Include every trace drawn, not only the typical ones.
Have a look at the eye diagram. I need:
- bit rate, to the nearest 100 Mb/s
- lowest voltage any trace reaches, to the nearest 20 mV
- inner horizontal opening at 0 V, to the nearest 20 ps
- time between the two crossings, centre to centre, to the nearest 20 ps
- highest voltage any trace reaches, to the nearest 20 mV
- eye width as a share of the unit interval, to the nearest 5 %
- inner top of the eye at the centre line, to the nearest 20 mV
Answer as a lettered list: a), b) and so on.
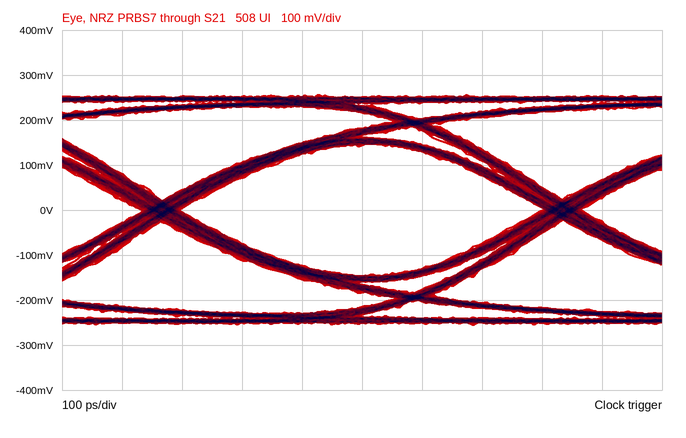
a) 1.5 Gb/s
b) -260 mV
c) 600 ps
d) 660 ps
e) 260 mV
f) 90 %
g) 140 mV
